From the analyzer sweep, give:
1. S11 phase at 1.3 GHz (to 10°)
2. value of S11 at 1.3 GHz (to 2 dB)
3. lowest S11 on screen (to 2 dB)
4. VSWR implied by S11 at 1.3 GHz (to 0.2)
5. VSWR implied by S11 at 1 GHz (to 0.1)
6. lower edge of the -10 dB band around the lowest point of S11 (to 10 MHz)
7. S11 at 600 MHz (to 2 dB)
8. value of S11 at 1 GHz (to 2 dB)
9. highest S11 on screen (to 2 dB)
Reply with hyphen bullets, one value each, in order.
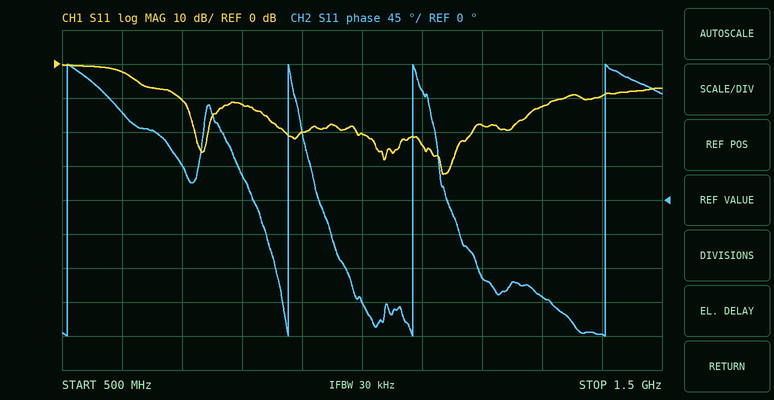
- -130°
- -12 dB
- -32 dB
- 1.6
- 1.2
- 700 MHz
- -2 dB
- -20 dB
- 0 dB
